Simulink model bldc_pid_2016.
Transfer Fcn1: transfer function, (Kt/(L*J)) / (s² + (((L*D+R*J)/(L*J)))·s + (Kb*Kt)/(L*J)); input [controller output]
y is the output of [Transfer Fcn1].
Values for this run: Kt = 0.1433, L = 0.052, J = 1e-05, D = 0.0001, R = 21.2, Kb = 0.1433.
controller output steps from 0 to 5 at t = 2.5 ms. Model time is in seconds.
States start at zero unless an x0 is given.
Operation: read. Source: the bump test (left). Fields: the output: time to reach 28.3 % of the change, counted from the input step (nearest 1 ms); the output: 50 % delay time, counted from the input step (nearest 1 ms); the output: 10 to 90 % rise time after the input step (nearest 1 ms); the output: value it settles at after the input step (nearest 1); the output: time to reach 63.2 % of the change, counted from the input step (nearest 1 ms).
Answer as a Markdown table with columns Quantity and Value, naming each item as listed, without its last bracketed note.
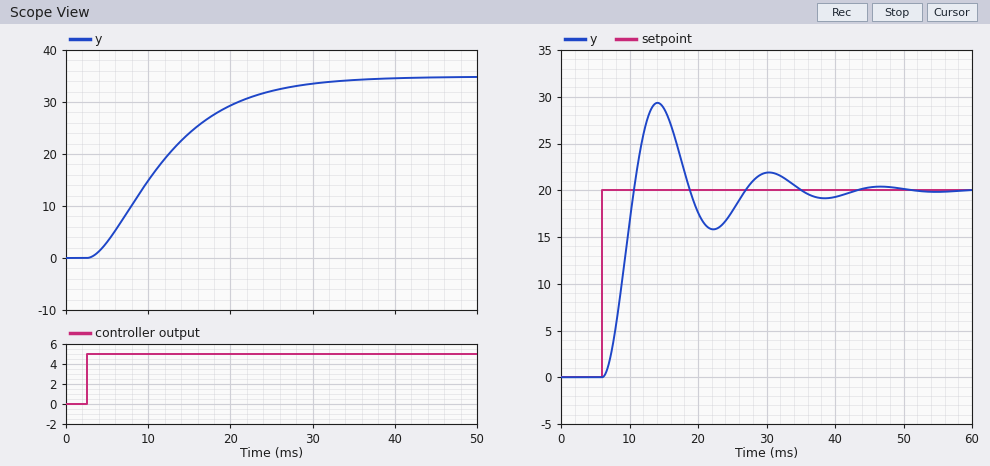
| Quantity | Value |
|---|---|
| the output: time to reach 28.3 % of the change, counted from the input step | 5 ms |
| the output: 50 % delay time, counted from the input step | 9 ms |
| the output: 10 to 90 % rise time after the input step | 18 ms |
| the output: value it settles at after the input step | 35 |
| the output: time to reach 63.2 % of the change, counted from the input step | 11 ms |
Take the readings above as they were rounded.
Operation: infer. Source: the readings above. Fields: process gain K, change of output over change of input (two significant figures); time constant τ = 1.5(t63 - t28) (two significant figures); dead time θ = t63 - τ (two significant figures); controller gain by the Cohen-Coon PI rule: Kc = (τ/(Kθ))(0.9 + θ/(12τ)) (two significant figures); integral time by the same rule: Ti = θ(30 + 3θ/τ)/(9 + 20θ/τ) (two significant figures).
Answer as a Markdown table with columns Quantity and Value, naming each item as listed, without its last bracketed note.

| Quantity | Value |
|---|---|
| process gain K, change of output over change of input | 7.0 |
| time constant τ = 1.5(t63 - t28) | 9.0 ms |
| dead time θ = t63 - τ | 2.0 ms |
| controller gain by the Cohen-Coon PI rule: Kc = (τ/(Kθ))(0.9 + θ/(12τ)) | 0.59 |
| integral time by the same rule: Ti = θ(30 + 3θ/τ)/(9 + 20θ/τ) | 4.6 ms |
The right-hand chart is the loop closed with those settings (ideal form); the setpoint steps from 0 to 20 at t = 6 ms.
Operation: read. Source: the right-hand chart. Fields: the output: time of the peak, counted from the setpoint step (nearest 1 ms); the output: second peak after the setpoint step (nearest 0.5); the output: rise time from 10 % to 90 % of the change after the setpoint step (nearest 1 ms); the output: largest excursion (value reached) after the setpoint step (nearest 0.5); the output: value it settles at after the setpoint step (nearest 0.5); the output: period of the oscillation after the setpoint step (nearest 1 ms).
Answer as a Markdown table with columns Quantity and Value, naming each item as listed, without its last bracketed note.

| Quantity | Value |
|---|---|
| the output: time of the peak, counted from the setpoint step | 8 ms |
| the output: second peak after the setpoint step | 22.0 |
| the output: rise time from 10 % to 90 % of the change after the setpoint step | 3 ms |
| the output: largest excursion (value reached) after the setpoint step | 29.5 |
| the output: value it settles at after the setpoint step | 20.0 |
| the output: period of the oscillation after the setpoint step | 16 ms |
